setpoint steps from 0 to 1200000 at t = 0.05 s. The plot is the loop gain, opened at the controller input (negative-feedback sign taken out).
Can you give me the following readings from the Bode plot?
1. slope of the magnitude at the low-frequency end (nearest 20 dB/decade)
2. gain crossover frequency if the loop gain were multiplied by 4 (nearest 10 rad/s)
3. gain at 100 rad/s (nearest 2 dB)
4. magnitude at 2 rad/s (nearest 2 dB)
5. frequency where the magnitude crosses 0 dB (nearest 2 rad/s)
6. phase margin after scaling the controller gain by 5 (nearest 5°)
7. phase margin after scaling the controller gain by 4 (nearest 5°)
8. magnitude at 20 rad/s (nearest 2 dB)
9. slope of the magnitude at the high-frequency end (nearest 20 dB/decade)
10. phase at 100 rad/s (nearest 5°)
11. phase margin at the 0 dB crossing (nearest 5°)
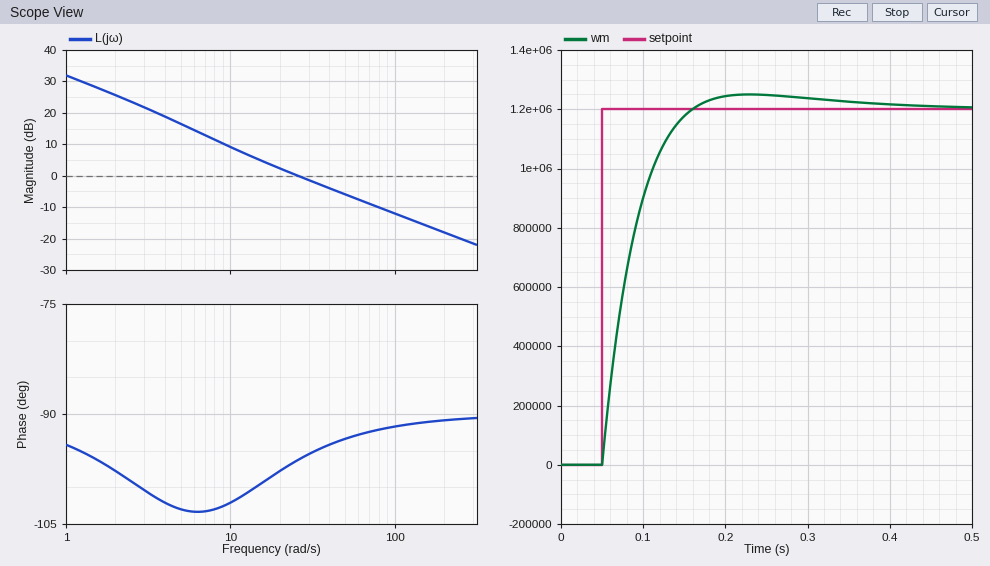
-20 dB/decade
100 rad/s
-12 dB
26 dB
26 rad/s
90°
90°
2 dB
-20 dB/decade
-90°
85°
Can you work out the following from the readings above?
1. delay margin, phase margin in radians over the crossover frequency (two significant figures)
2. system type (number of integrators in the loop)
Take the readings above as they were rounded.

0.057 s
1
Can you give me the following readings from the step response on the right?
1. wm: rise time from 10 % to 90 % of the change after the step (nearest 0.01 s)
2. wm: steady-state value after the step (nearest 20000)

0.07 s
1200000
